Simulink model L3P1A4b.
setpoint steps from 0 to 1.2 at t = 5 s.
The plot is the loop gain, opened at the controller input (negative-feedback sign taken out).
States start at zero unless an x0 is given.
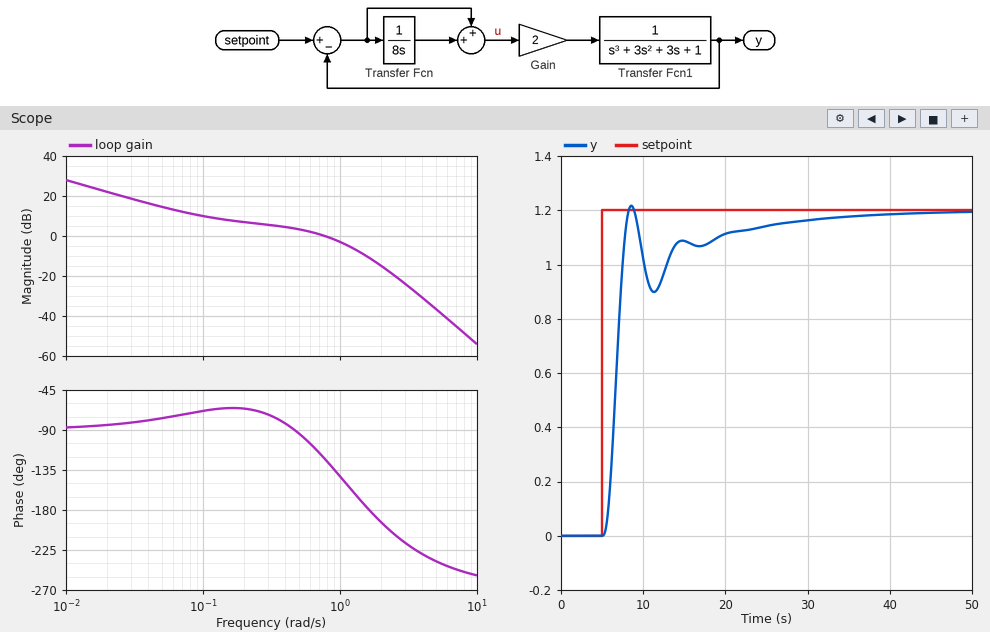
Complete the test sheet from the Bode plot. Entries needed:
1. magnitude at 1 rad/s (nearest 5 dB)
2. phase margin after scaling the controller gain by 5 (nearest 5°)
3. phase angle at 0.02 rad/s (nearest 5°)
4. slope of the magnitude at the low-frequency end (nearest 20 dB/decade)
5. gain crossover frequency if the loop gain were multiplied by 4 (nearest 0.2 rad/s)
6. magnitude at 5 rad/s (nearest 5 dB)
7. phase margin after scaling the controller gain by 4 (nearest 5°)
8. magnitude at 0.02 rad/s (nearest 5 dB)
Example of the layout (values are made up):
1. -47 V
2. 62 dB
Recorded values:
1. -5 dB
2. -10°
3. -85°
4. -20 dB/decade
5. 1.8 rad/s
6. -35 dB
7. -5°
8. 20 dB
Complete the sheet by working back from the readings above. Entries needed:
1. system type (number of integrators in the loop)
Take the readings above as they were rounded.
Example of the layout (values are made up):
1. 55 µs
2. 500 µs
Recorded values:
1. 1
